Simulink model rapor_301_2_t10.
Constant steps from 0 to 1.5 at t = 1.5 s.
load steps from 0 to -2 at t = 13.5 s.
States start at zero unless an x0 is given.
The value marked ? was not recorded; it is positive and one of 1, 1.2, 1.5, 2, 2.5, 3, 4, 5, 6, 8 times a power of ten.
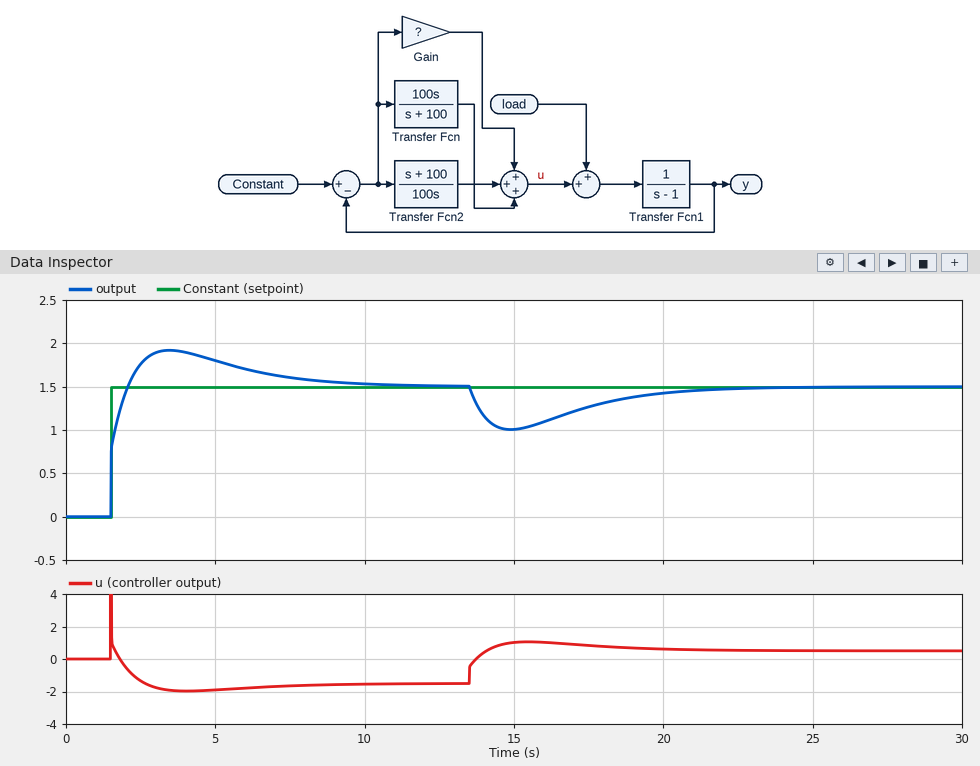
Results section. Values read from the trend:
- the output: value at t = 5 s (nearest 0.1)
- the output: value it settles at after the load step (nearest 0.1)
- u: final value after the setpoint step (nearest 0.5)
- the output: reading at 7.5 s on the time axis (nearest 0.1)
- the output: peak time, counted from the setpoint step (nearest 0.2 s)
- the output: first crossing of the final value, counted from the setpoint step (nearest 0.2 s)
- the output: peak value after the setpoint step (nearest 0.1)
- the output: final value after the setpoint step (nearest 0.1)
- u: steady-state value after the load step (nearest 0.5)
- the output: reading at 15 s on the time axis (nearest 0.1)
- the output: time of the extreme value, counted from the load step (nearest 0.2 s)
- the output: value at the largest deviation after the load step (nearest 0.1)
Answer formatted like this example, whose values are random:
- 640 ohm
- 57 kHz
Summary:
- 1.8
- 1.5
- -1.5
- 1.6
- 2.0 s
- 0.6 s
- 1.9
- 1.5
- 0.5
- 1.0
- 1.4 s
- 1.0
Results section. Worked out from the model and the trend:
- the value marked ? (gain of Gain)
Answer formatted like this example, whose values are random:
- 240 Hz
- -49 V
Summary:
- 4
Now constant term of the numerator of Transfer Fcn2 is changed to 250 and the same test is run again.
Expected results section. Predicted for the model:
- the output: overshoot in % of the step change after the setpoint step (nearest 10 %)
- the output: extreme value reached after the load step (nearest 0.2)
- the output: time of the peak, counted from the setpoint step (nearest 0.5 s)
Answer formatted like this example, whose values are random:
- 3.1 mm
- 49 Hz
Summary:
- 30 %
- 1.0
- 1.5 s
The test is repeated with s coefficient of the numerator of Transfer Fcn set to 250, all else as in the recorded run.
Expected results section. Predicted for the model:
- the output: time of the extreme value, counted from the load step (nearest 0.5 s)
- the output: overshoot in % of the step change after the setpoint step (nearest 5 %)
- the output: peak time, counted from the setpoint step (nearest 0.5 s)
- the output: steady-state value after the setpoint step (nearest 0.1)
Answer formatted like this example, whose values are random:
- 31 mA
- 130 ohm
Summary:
- 2.0 s
- 25 %
- 2.5 s
- 1.5
